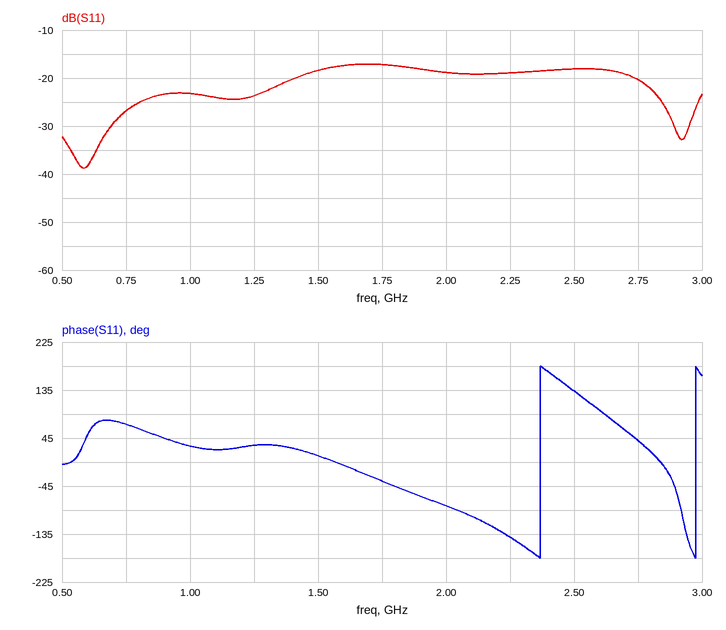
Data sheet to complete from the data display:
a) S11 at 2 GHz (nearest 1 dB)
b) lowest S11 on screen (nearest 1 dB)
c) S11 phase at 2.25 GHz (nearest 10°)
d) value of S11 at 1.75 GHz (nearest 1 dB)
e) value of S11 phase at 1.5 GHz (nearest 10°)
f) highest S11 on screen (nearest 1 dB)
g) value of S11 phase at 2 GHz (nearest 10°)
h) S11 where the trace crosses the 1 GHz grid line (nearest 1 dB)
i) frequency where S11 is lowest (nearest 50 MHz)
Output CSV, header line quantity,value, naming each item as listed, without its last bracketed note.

quantity,value
S11 at 2 GHz,-19 dB
lowest S11 on screen,-39 dB
S11 phase at 2.25 GHz,-140°
value of S11 at 1.75 GHz,-17 dB
value of S11 phase at 1.5 GHz,10°
highest S11 on screen,-17 dB
value of S11 phase at 2 GHz,-80°
S11 where the trace crosses the 1 GHz grid line,-23 dB
frequency where S11 is lowest,600 MHz
